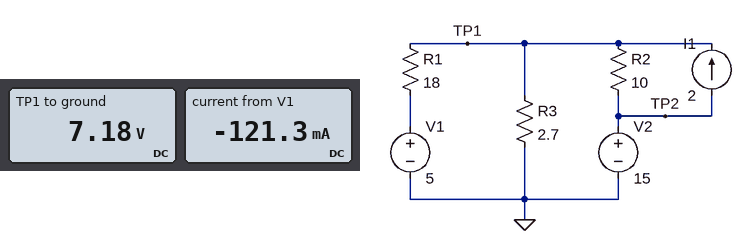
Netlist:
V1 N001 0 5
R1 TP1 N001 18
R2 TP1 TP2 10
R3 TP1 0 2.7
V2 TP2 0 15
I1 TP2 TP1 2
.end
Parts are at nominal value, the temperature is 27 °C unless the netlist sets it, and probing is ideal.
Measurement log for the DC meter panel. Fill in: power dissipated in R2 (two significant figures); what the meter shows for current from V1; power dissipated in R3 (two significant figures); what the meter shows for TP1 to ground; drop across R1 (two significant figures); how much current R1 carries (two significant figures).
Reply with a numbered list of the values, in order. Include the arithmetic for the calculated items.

1. (15 V - 7.18 V)^2 / 10 Ω = 6.1 W
2. -121.3 mA
3. (7.18 V)^2 / 2.7 Ω = 19 W
4. 7.18 V
5. 7.18 V - 5 V = 2.2 V
6. (7.18 V - 5 V) / 18 Ω = 120 mA
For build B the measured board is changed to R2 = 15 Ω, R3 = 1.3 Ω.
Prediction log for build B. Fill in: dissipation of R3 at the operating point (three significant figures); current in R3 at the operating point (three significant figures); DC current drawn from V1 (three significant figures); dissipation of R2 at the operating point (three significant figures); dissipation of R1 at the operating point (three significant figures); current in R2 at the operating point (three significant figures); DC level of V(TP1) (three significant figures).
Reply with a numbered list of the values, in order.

1. 10.4 W
2. 2.83 A
3. 73.5 mA
4. 8.55 W
5. 97.3 mW
6. 755 mA
7. 3.68 V
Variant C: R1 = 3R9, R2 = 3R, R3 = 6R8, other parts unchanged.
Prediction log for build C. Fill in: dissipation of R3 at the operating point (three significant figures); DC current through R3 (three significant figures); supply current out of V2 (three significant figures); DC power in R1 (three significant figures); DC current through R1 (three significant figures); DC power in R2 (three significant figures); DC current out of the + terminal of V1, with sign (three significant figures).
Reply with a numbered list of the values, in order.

1. 18.6 W
2. 1.65 A
3. 3.25 A
4. 9.99 W
5. 1.60 A
6. 4.71 W
7. -1.60 A
